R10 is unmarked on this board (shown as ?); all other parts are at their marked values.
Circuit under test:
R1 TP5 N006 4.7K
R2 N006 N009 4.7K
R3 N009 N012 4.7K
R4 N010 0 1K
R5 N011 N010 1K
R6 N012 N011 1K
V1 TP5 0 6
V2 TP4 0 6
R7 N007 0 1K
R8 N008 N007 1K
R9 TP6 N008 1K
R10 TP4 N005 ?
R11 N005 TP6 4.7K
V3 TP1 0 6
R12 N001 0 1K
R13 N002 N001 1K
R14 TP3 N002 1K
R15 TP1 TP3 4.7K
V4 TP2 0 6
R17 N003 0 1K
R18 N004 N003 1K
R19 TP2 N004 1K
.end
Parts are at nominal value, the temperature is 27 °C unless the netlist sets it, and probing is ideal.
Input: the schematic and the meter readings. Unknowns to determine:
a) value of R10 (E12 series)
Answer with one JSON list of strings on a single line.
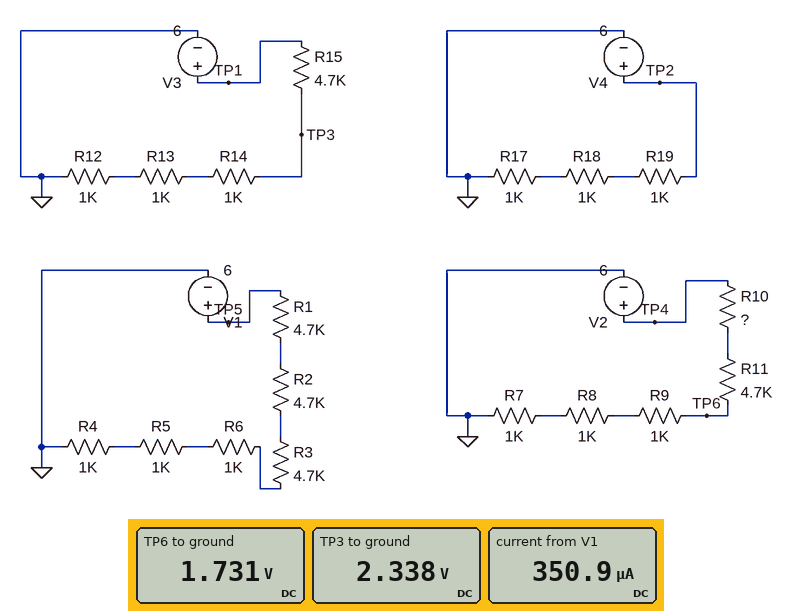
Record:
["2.7 kΩ"]
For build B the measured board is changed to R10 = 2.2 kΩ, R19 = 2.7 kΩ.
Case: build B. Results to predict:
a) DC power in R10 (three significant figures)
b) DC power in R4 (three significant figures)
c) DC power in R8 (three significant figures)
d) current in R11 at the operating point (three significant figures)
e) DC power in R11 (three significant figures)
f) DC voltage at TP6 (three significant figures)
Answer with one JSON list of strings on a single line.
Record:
["808 µW", "123 µW", "367 µW", "606 µA", "1.73 mW", "1.82 V"]
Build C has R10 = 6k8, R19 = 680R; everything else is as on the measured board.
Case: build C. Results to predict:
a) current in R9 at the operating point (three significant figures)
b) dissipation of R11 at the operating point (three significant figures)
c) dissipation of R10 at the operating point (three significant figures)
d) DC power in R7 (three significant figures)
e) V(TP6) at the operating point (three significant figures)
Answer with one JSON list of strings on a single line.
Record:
["414 µA", "805 µW", "1.16 mW", "171 µW", "1.24 V"]
